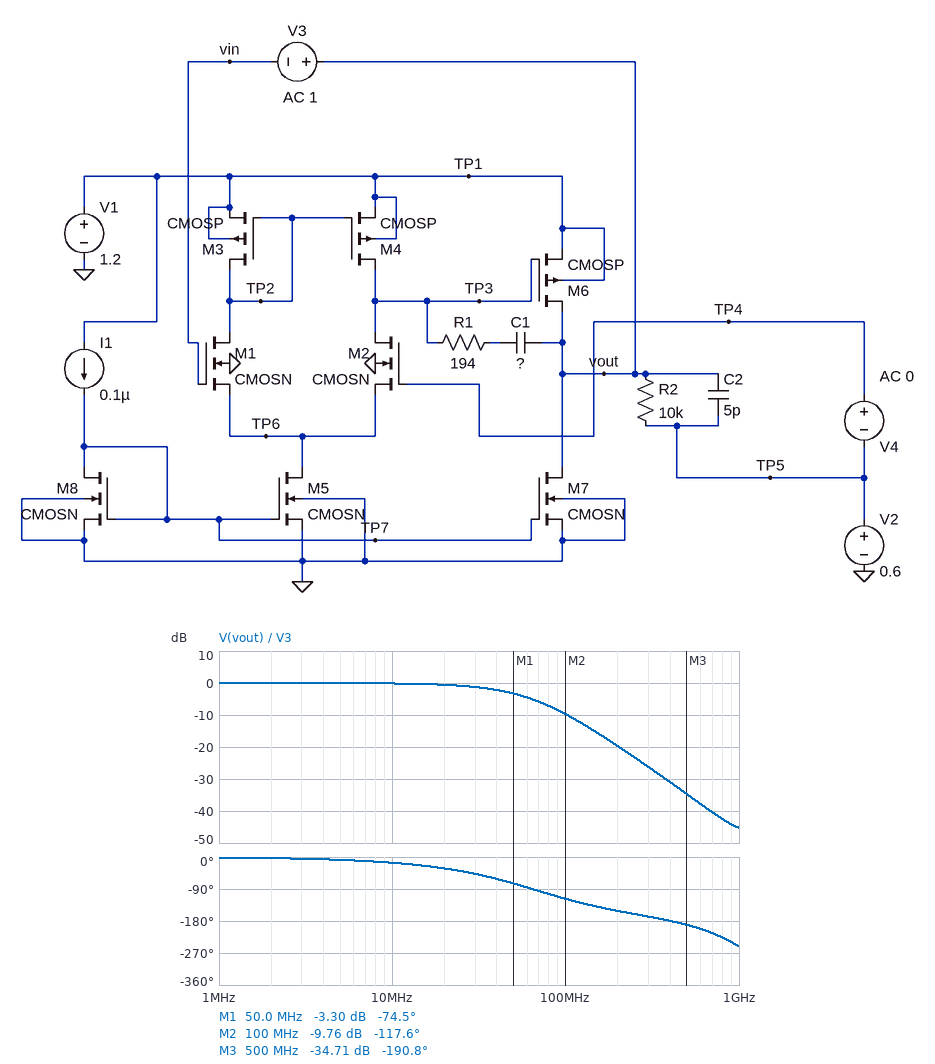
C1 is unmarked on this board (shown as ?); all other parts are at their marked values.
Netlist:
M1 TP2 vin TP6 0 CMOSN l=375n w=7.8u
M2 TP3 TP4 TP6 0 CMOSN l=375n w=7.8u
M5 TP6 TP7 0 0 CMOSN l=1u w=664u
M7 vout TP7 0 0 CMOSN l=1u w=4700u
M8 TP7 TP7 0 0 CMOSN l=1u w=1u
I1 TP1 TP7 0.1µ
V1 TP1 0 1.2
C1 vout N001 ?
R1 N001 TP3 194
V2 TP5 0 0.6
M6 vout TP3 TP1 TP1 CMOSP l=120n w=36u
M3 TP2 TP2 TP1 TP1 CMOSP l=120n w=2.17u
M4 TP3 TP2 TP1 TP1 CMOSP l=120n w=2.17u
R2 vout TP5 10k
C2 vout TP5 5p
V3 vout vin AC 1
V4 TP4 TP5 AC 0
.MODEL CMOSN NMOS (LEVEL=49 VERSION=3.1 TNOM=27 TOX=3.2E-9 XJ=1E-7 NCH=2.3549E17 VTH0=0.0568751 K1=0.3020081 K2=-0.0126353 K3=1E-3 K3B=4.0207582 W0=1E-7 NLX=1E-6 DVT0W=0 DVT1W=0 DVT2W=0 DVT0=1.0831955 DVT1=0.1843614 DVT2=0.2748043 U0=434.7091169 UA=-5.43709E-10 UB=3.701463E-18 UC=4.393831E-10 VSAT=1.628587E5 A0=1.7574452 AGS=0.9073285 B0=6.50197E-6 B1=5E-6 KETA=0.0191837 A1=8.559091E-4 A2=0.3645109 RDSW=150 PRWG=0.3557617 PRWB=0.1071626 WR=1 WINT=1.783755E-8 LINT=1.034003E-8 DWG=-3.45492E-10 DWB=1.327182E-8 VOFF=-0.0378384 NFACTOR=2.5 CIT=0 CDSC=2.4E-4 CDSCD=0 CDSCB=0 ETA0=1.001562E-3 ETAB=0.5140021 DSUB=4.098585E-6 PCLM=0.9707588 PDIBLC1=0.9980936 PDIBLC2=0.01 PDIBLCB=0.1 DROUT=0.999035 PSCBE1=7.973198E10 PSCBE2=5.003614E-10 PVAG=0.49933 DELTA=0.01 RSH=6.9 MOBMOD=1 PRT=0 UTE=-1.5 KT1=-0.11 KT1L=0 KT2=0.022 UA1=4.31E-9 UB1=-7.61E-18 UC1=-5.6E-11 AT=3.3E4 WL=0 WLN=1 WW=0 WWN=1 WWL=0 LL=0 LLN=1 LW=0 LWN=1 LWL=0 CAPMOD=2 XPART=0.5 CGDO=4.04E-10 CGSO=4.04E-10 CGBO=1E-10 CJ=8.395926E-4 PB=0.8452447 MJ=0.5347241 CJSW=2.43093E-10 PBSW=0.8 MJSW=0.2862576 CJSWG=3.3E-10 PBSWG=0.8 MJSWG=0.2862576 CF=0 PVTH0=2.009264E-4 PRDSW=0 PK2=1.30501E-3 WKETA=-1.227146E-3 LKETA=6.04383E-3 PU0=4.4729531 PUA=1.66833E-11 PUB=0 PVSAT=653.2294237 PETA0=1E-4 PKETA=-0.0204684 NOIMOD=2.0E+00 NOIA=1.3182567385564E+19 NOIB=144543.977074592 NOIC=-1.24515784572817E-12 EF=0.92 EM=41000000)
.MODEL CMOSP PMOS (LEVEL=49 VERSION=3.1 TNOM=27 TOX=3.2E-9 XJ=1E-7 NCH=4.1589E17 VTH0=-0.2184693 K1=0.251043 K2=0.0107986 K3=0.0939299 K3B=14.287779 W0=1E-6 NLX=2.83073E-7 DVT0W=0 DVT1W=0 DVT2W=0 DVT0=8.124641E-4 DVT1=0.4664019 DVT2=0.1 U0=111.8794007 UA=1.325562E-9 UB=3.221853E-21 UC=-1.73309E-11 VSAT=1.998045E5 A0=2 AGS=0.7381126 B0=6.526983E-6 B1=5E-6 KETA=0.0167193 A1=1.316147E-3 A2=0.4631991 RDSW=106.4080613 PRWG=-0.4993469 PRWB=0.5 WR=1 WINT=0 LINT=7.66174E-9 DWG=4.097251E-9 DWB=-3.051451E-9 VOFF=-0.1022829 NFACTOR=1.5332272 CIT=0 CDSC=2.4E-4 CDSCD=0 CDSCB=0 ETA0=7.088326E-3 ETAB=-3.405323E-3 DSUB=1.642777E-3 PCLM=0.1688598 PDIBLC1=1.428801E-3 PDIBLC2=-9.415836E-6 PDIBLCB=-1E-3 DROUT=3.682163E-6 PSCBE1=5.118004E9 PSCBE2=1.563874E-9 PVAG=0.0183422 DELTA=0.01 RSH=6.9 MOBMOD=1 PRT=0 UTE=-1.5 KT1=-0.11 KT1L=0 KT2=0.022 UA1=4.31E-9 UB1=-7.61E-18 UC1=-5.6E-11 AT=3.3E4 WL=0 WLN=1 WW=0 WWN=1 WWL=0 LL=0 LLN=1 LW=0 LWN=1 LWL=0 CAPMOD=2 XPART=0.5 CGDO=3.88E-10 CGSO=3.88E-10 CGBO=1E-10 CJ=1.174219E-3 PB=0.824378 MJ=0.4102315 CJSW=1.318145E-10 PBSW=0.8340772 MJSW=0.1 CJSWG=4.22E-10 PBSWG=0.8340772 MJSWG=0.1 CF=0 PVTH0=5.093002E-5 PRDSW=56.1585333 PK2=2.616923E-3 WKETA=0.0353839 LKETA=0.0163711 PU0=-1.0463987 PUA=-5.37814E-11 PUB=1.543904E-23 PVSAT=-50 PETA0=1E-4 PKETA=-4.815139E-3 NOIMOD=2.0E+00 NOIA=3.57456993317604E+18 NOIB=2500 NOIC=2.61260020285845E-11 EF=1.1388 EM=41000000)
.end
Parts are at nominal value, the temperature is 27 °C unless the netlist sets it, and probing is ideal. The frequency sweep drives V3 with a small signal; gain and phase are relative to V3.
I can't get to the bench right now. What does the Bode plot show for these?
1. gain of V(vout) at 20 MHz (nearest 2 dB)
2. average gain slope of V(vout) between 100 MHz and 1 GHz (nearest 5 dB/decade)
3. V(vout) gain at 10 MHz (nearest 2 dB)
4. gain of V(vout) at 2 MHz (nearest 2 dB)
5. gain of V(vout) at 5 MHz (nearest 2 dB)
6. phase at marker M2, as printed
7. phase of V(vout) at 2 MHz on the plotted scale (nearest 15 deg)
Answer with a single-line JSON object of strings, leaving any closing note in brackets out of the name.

{"gain of V(vout) at 20 MHz": "0 dB", "average gain slope of V(vout) between 100 MHz and 1 GHz": "-35 dB/decade", "V(vout) gain at 10 MHz": "0 dB", "gain of V(vout) at 2 MHz": "0 dB", "gain of V(vout) at 5 MHz": "0 dB", "phase at marker M2, as printed": "-117.6 deg", "phase of V(vout) at 2 MHz on the plotted scale": "0 deg"}
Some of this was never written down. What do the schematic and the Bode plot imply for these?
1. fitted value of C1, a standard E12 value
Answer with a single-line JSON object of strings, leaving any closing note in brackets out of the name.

{"fitted value of C1, a standard E12 value": "2.7 pF"}
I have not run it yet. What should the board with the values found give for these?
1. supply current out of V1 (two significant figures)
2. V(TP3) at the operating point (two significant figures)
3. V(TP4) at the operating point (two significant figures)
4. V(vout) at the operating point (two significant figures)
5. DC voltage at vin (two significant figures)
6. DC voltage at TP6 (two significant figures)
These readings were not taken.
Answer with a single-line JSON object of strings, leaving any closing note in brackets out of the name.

{"supply current out of V1": "610 µA", "V(TP3) at the operating point": "590 mV", "V(TP4) at the operating point": "600 mV", "V(vout) at the operating point": "600 mV", "DC voltage at vin": "600 mV", "DC voltage at TP6": "190 mV"}
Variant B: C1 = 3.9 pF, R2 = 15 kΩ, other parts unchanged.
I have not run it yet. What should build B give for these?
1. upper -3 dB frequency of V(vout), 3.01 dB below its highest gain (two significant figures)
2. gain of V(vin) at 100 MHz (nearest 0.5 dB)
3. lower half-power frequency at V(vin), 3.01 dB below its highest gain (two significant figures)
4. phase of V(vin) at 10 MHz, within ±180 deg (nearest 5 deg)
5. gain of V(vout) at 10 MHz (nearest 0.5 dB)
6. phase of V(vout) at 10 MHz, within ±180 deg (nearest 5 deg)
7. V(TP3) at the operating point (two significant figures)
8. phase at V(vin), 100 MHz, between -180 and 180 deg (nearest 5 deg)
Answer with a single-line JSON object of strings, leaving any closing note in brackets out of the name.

{"upper -3 dB frequency of V(vout), 3.01 dB below its highest gain": "31 MHz", "gain of V(vin) at 100 MHz": "1.0 dB", "lower half-power frequency at V(vin), 3.01 dB below its highest gain": "25 MHz", "phase of V(vin) at 10 MHz, within ±180 deg": "-110 deg", "gain of V(vout) at 10 MHz": "-0.5 dB", "phase of V(vout) at 10 MHz, within ±180 deg": "-25 deg", "V(TP3) at the operating point": "590 mV", "phase at V(vin), 100 MHz, between -180 and 180 deg": "-170 deg"}
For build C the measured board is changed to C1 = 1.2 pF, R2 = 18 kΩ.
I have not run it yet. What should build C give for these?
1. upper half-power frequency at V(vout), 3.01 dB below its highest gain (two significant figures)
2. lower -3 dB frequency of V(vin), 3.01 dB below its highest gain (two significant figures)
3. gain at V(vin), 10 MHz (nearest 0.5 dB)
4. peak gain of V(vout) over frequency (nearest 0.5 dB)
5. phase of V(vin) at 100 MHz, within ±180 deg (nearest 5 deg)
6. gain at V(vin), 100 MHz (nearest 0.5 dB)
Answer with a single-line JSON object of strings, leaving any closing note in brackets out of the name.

{"upper half-power frequency at V(vout), 3.01 dB below its highest gain": "110 MHz", "lower -3 dB frequency of V(vin), 3.01 dB below its highest gain": "65 MHz", "gain at V(vin), 10 MHz": "-18.0 dB", "peak gain of V(vout) over frequency": "0.5 dB", "phase of V(vin) at 100 MHz, within ±180 deg": "-145 deg", "gain at V(vin), 100 MHz": "2.5 dB"}
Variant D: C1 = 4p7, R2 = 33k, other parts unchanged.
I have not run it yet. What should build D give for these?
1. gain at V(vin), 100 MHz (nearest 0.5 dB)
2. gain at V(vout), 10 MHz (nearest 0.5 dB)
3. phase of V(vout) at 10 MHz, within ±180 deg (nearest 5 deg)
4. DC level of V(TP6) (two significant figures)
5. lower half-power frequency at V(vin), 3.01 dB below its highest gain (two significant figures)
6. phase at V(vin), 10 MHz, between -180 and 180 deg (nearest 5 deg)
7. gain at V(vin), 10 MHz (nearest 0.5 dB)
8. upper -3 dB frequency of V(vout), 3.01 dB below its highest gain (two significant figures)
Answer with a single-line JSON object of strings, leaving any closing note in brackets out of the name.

{"gain at V(vin), 100 MHz": "1.0 dB", "gain at V(vout), 10 MHz": "-0.5 dB", "phase of V(vout) at 10 MHz, within ±180 deg": "-25 deg", "DC level of V(TP6)": "190 mV", "lower half-power frequency at V(vin), 3.01 dB below its highest gain": "21 MHz", "phase at V(vin), 10 MHz, between -180 and 180 deg": "-110 deg", "gain at V(vin), 10 MHz": "-7.0 dB", "upper -3 dB frequency of V(vout), 3.01 dB below its highest gain": "25 MHz"}
